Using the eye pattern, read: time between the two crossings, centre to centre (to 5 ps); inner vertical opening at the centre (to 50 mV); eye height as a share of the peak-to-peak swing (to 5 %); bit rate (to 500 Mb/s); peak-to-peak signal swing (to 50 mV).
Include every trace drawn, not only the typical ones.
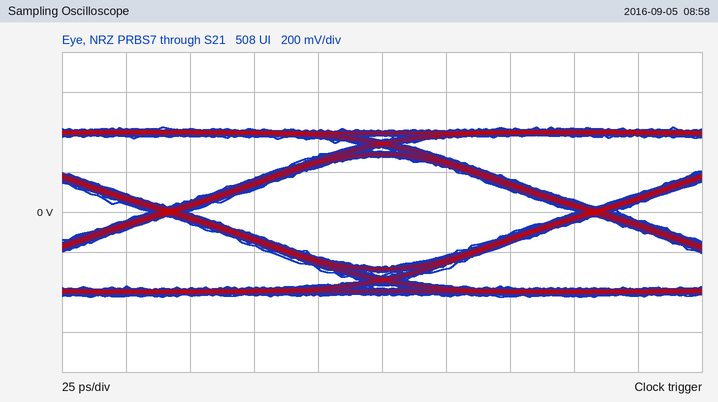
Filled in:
165 ps
550 mV
65 %
6.0 Gb/s
850 mV
